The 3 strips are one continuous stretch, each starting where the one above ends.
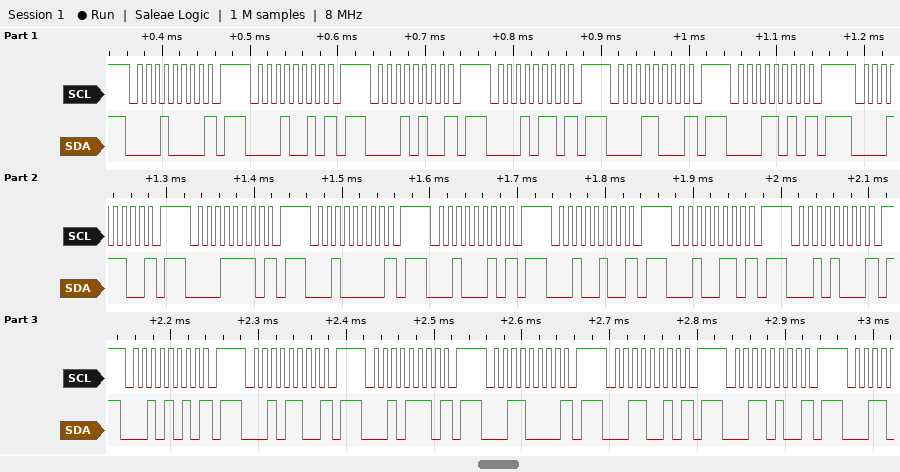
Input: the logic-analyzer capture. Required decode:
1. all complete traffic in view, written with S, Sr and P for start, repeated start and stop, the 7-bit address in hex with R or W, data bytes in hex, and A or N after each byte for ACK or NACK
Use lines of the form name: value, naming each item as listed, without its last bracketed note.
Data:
all complete traffic in view, written with S, Sr and P for start, repeated start and stop, the 7-bit address in hex with R or W, data bytes in hex, and A or N after each byte for ACK or NACK: S 08W N P S 09W N P S 0AW N P S 0BW N P S 0CW N P S 0DW N P S 0EW N P S 0FW N P S 10W N P S 11W N P S 12W N P S 13W N P S 14W N P S 15W N P S 16W N P S 17W N P S 18W N P S 19W N P S 1AW N P
